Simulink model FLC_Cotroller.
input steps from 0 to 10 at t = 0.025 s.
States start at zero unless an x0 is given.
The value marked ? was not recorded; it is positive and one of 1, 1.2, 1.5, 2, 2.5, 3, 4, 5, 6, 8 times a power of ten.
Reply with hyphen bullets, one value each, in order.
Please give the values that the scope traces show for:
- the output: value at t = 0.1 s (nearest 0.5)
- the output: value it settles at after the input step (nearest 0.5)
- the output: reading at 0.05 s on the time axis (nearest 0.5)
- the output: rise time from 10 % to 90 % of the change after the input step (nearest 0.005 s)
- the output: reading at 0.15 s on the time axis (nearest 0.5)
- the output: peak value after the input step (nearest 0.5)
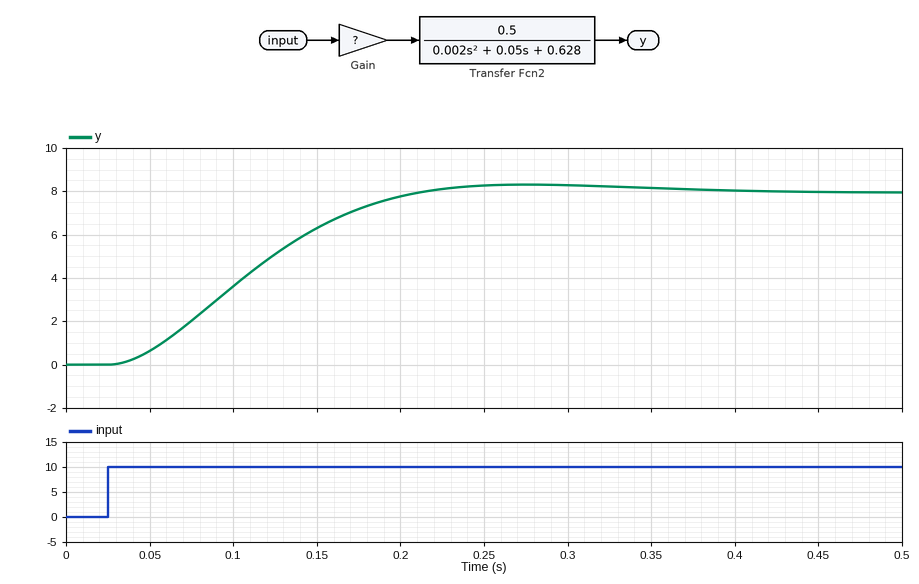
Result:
- 3.5
- 8.0
- 0.5
- 0.120 s
- 6.5
- 8.5
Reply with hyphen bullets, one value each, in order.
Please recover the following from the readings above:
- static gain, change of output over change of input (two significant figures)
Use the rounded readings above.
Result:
- 0.80
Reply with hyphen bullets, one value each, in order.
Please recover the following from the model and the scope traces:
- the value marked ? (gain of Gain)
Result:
- 1
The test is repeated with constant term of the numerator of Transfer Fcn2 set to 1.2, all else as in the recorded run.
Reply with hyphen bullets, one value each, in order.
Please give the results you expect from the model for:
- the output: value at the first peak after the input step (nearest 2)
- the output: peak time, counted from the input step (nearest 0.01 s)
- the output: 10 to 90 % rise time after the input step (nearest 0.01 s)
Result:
- 20
- 0.25 s
- 0.12 s
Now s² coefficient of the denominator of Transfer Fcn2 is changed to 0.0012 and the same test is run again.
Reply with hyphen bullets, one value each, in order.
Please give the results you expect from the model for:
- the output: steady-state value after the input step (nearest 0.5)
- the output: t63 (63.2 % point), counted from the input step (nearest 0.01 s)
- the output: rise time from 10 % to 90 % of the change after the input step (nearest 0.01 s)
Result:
- 8.0
- 0.09 s
- 0.13 s
